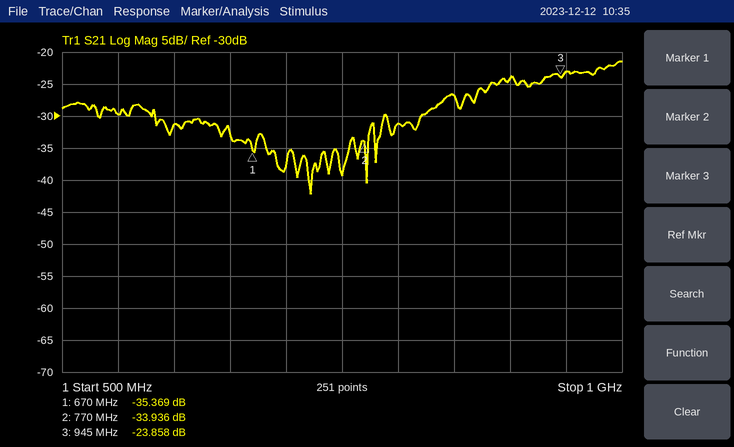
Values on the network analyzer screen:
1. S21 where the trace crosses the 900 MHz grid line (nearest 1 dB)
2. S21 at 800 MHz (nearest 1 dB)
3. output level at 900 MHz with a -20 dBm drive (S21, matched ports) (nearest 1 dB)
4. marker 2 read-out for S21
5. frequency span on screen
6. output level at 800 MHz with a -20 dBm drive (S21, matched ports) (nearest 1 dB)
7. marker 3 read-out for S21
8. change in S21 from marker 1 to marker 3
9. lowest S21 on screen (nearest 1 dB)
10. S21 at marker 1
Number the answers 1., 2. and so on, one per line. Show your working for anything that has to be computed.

1. -24 dB
2. -31 dB
3. -20 dBm + (-24 dB) = -44 dBm
4. -33.936 dB
5. 500 MHz
6. -20 dBm + (-31 dB) = -51 dBm
7. -23.858 dB
8. -23.858 − (-35.369) = 11.511 dB
9. -42 dB
10. -35.369 dB
